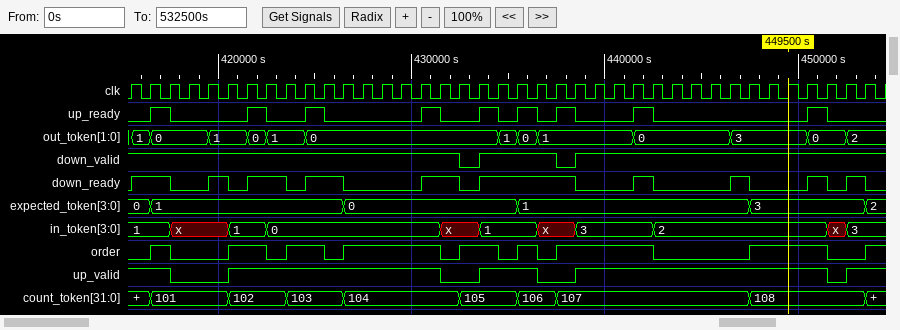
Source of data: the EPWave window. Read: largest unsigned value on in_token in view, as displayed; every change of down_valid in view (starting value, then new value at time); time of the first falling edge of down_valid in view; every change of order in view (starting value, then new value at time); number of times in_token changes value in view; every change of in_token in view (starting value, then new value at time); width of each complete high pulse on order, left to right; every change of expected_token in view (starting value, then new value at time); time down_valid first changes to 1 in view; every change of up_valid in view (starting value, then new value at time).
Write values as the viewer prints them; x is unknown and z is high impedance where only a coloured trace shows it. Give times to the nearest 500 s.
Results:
3
1, 0 at 432500 s, 1 at 433500 s, 0 at 437500 s, 1 at 438500 s
432500 s
0, 1 at 416500 s, 0 at 417500 s, 1 at 420500 s, 0 at 422500 s, 1 at 423500 s, 0 at 425500 s, 1 at 426500 s, 0 at 431500 s, 1 at 432500 s, 0 at 434500 s, 1 at 435500 s, 0 at 436500 s, 1 at 437500 s, 0 at 442500 s, 1 at 447500 s, 0 at 451500 s, 1 at 453500 s
10
1, x at 417500 s, 1 at 420500 s, 0 at 422500 s, x at 431500 s, 1 at 433500 s, x at 436500 s, 3 at 438500 s, 2 at 442500 s, x at 451500 s, 3 at 452500 s
1000 s, 2000 s, 2000 s, 5000 s, 2000 s, 1000 s, 5000 s, 4000 s
0, 1 at 416500 s, 0 at 426500 s, 1 at 435500 s, 3 at 447500 s, 2 at 453500 s
433500 s
1, 0 at 417500 s, 1 at 420500 s, 0 at 431500 s, 1 at 433500 s, 0 at 436500 s, 1 at 438500 s, 0 at 451500 s, 1 at 452500 s
